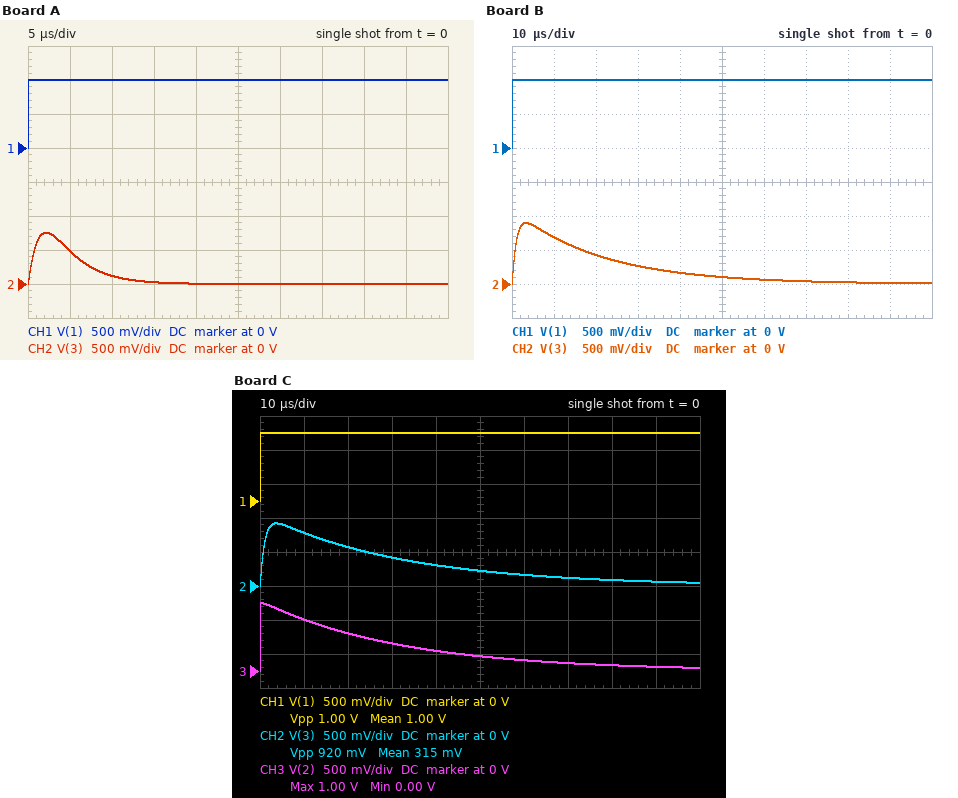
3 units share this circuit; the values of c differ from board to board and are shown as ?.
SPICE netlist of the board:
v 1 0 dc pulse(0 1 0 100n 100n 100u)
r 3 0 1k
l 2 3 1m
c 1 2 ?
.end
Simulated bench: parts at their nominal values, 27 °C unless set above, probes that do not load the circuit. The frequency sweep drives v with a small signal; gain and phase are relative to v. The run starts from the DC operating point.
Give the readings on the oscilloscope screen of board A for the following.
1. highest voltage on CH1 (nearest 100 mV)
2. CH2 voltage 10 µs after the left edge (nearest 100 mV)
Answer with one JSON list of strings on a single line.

["1.0 V", "100 mV"]
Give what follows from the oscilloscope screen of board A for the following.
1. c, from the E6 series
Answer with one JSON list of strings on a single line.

["4.7 nF"]
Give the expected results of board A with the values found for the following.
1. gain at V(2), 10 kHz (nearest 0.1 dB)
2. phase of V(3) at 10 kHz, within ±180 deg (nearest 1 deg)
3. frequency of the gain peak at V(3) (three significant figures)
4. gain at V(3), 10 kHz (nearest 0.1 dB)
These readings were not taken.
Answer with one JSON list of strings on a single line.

["-10.8 dB", "73 deg", "73.4 kHz", "-10.8 dB"]
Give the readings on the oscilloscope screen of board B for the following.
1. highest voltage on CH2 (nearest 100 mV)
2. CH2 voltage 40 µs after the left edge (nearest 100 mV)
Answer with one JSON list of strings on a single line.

["900 mV", "200 mV"]
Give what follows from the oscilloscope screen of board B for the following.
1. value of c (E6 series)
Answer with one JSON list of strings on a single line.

["22 nF"]
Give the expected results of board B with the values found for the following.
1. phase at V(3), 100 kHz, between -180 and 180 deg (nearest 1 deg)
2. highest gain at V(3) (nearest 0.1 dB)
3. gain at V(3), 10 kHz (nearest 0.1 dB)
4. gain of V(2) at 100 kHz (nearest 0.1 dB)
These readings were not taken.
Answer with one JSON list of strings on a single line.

["-29 deg", "0 dB", "-1.6 dB", "0.3 dB"]
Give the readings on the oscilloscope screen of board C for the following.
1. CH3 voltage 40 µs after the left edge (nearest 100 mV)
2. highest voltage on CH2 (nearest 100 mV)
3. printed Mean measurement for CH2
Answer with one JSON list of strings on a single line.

["300 mV", "900 mV", "315 mV"]
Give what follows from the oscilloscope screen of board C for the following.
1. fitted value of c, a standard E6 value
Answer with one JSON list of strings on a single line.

["33 nF"]
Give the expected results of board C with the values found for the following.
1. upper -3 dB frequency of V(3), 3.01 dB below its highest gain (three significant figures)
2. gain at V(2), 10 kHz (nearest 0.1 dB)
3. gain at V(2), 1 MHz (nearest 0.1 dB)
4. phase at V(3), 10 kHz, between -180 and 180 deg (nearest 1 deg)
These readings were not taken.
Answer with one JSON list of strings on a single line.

["164 kHz", "-0.7 dB", "0 dB", "23 deg"]
